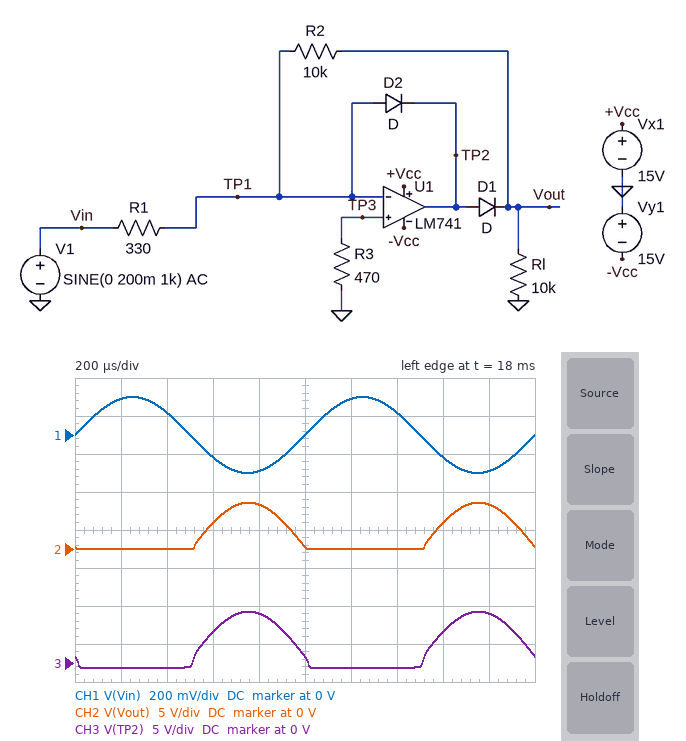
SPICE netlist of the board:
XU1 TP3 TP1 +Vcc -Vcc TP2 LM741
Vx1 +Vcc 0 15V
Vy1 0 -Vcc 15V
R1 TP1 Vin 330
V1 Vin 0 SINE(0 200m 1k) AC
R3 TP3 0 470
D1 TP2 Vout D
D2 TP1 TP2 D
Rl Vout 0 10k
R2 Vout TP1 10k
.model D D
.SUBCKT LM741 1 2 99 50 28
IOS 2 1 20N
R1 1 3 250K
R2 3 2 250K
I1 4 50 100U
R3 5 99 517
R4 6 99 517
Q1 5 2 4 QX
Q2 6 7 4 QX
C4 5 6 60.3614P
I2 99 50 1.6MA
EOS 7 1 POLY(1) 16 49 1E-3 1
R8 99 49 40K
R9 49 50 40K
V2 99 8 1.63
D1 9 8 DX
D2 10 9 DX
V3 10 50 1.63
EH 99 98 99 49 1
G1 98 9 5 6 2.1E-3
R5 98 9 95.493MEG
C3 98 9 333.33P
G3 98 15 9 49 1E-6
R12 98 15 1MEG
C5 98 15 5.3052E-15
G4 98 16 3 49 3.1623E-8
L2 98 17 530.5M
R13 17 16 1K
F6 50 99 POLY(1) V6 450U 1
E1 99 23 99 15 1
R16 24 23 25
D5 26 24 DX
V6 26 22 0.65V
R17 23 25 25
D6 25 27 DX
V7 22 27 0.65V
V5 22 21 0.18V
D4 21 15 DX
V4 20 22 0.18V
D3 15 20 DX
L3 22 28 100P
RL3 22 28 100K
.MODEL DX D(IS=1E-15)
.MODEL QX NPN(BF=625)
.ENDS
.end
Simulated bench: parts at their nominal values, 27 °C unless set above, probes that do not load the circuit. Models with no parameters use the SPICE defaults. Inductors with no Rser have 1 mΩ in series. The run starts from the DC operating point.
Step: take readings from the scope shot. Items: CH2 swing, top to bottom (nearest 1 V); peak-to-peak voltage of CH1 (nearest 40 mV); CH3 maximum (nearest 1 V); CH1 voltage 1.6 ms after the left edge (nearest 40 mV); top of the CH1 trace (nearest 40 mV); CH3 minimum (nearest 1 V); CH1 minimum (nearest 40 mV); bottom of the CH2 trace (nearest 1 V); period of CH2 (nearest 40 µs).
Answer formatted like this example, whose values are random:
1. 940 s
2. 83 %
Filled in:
1. 6 V
2. 400 mV
3. 7 V
4. -120 mV
5. 200 mV
6. -1 V
7. -200 mV
8. 0 V
9. 1.00 ms
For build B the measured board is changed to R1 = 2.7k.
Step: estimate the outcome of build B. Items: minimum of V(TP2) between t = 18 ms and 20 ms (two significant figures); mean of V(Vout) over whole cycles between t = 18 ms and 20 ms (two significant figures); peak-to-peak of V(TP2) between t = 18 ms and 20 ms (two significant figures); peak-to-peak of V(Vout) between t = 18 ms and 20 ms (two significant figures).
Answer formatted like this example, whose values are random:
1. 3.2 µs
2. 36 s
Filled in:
1. -590 mV
2. 240 mV
3. 1.9 V
4. 750 mV
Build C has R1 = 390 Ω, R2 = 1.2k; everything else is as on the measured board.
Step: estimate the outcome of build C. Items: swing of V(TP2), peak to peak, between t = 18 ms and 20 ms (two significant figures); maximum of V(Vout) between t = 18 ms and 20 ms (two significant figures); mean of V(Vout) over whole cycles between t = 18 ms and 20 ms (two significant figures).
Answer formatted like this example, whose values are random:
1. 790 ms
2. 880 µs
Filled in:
1. 1.9 V
2. 620 mV
3. 200 mV
